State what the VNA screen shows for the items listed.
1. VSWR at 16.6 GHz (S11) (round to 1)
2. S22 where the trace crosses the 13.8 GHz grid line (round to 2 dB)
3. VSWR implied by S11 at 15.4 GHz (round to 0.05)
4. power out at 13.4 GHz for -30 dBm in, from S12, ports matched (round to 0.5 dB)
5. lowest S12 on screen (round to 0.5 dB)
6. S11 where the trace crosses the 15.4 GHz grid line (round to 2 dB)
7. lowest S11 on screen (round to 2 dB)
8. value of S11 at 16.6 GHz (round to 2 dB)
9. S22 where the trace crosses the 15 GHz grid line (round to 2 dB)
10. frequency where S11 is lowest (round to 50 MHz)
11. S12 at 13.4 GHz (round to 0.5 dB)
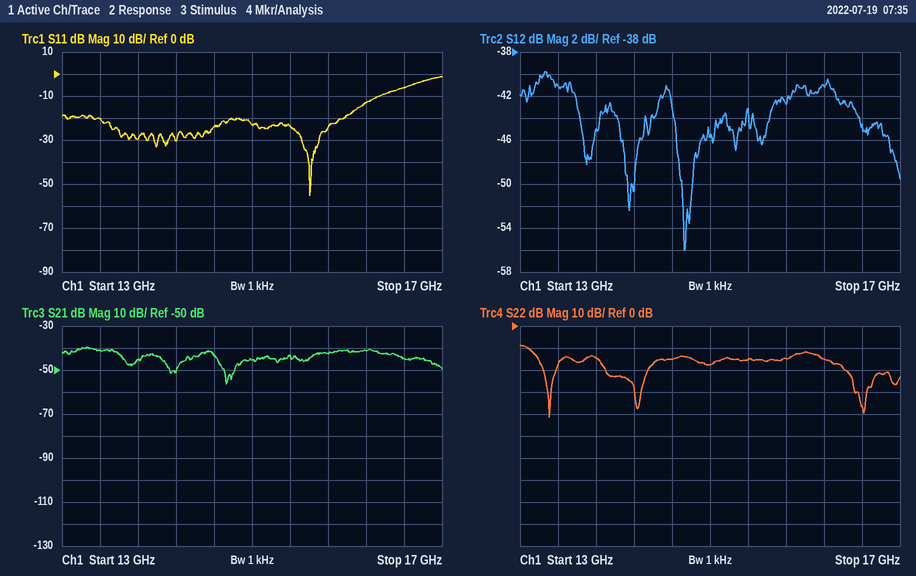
3
-14 dB
1.15
-71.0 dBm
-56.0 dB
-24 dB
-56 dB
-6 dB
-18 dB
15.60 GHz
-41.0 dB
